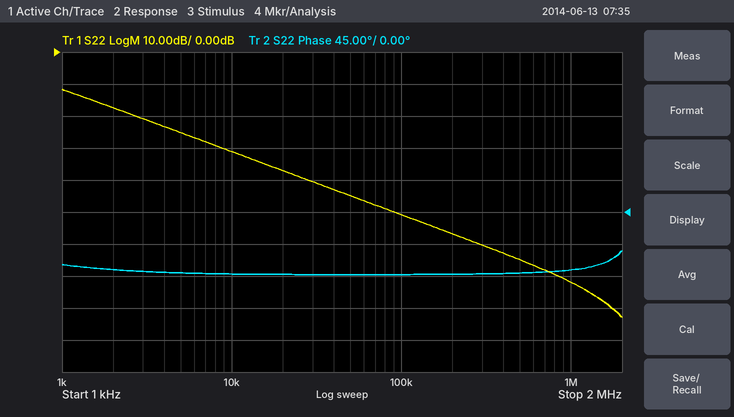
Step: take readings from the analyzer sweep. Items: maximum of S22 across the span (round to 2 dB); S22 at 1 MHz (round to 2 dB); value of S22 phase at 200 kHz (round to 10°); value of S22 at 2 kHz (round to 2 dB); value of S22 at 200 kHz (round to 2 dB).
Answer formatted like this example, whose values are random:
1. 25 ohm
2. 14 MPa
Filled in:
1. -12 dB
2. -72 dB
3. -90°
4. -18 dB
5. -56 dB
